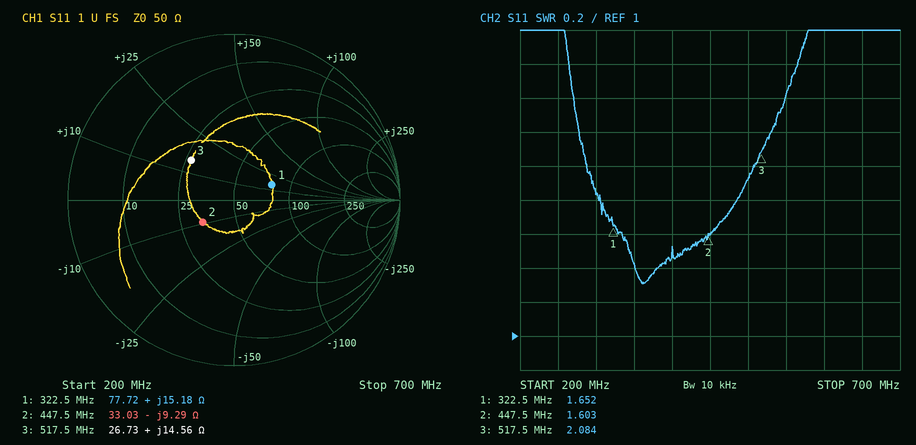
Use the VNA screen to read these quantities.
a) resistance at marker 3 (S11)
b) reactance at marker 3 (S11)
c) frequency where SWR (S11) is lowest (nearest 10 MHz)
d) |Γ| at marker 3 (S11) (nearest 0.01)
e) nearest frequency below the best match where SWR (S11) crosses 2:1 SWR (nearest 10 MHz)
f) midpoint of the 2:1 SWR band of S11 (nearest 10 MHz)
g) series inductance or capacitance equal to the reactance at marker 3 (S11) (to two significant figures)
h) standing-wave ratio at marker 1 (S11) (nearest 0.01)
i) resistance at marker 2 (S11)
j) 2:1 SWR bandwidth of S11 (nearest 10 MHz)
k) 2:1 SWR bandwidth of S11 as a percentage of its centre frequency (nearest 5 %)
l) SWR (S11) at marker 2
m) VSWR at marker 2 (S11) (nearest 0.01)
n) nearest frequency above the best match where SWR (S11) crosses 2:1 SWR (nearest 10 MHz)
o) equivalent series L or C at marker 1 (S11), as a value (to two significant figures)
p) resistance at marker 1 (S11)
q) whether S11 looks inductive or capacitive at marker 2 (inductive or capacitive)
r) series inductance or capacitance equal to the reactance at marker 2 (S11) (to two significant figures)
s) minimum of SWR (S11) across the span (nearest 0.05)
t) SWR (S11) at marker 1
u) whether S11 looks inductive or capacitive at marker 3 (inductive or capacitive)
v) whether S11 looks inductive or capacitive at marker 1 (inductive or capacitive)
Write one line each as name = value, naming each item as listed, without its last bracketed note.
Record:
resistance at marker 3 = 26.73 Ω
reactance at marker 3 = +14.56 Ω
frequency where SWR (S11) is lowest = 360 MHz
|Γ| at marker 3 (S11) = 0.35
nearest frequency below the best match where SWR (S11) crosses 2:1 SWR = 290 MHz
midpoint of the 2:1 SWR band of S11 = 400 MHz
series inductance or capacitance equal to the reactance at marker 3 (S11) = 4.5 nH
standing-wave ratio at marker 1 (S11) = 1.65
resistance at marker 2 = 33.03 Ω
2:1 SWR bandwidth of S11 = 220 MHz
2:1 SWR bandwidth of S11 as a percentage of its centre frequency = 55 %
SWR (S11) at marker 2 = 1.603
VSWR at marker 2 (S11) = 1.60
nearest frequency above the best match where SWR (S11) crosses 2:1 SWR = 510 MHz
equivalent series L or C at marker 1 (S11), as a value = 7.5 nH
resistance at marker 1 = 77.72 Ω
whether S11 looks inductive or capacitive at marker 2 = capacitive
series inductance or capacitance equal to the reactance at marker 2 (S11) = 38 pF
minimum of SWR (S11) across the span = 1.30
SWR (S11) at marker 1 = 1.652
whether S11 looks inductive or capacitive at marker 3 = inductive
whether S11 looks inductive or capacitive at marker 1 = inductive
